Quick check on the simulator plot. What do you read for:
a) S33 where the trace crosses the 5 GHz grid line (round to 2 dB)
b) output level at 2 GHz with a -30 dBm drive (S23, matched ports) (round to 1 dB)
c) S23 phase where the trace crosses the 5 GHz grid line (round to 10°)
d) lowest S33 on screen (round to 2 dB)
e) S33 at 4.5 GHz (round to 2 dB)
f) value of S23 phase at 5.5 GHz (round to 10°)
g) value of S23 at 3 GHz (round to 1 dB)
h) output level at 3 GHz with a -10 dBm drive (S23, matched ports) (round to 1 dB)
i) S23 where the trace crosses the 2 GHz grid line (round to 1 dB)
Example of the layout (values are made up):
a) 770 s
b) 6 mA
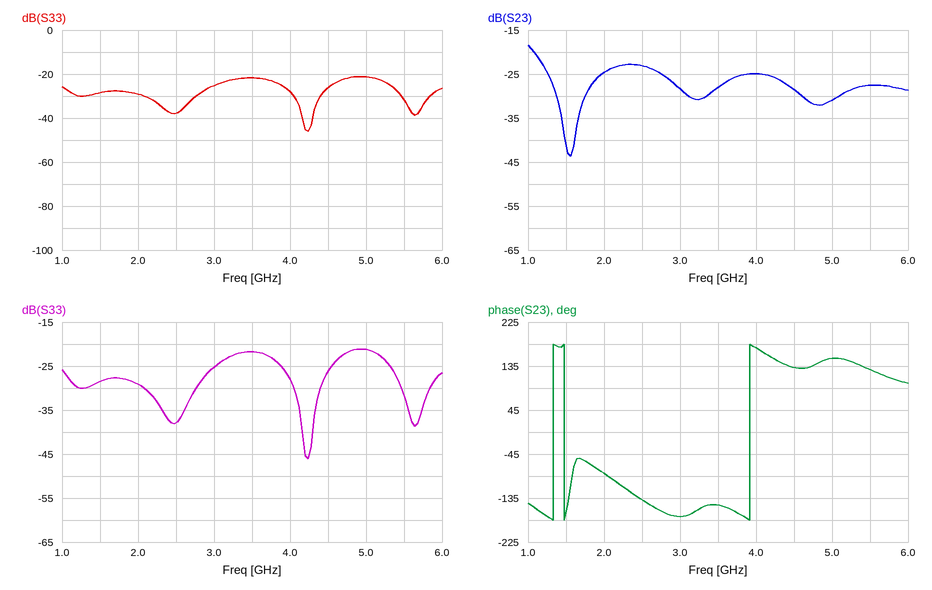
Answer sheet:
a) -22 dB
b) -55 dBm
c) 150°
d) -46 dB
e) -26 dB
f) 130°
g) -28 dB
h) -38 dBm
i) -25 dB
